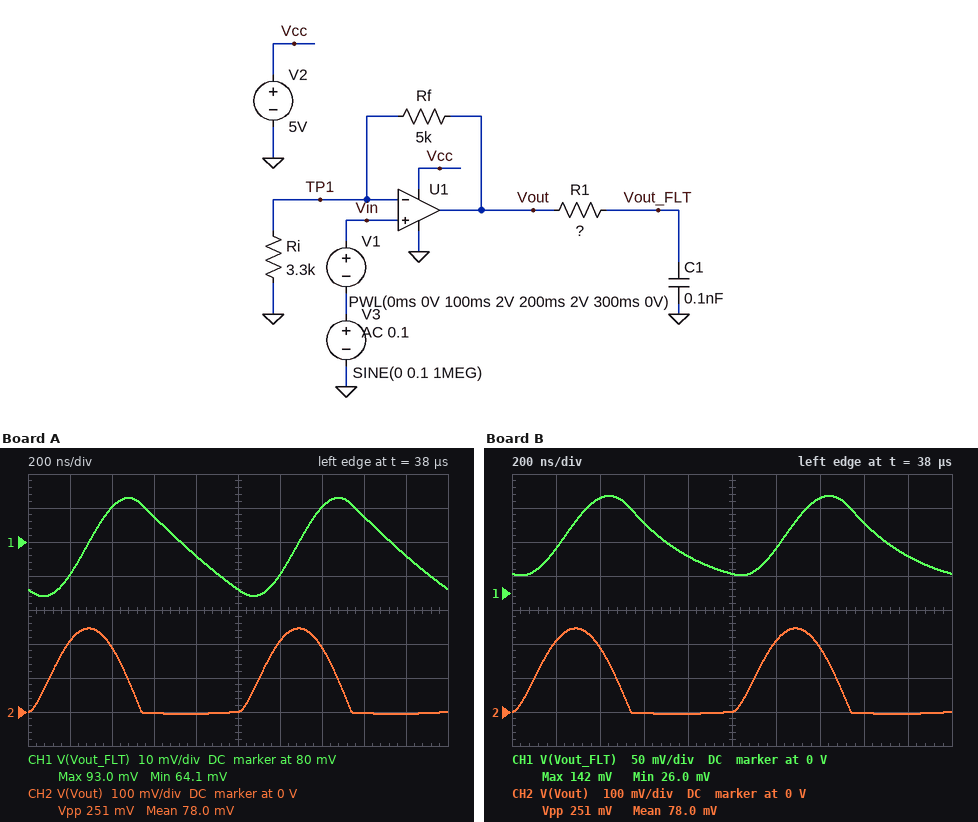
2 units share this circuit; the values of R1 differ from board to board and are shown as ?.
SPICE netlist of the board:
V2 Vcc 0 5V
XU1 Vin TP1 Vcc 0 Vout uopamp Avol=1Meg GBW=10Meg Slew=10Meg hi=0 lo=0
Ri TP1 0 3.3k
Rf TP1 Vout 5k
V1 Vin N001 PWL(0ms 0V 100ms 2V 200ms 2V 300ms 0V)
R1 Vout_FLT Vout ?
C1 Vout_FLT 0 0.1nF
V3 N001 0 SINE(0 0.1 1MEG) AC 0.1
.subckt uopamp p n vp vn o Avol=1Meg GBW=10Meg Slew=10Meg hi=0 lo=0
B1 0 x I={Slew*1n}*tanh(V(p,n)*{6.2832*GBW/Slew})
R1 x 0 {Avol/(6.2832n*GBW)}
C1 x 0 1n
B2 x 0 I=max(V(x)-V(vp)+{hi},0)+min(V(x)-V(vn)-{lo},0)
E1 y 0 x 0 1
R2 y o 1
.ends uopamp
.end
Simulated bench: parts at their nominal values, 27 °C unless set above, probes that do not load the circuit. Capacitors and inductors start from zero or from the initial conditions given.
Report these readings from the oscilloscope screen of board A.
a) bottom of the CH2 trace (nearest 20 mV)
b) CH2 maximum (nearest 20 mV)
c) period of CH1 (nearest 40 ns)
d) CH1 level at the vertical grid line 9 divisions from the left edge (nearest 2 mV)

0 V
240 mV
1.00 µs
76 mV
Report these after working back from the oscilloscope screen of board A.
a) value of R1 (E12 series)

15 kΩ
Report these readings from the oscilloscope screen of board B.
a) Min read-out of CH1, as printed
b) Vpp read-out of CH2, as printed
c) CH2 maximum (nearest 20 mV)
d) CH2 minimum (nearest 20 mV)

26.0 mV
251 mV
240 mV
0 V
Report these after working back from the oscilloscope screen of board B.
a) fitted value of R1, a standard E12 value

3.3 kΩ
